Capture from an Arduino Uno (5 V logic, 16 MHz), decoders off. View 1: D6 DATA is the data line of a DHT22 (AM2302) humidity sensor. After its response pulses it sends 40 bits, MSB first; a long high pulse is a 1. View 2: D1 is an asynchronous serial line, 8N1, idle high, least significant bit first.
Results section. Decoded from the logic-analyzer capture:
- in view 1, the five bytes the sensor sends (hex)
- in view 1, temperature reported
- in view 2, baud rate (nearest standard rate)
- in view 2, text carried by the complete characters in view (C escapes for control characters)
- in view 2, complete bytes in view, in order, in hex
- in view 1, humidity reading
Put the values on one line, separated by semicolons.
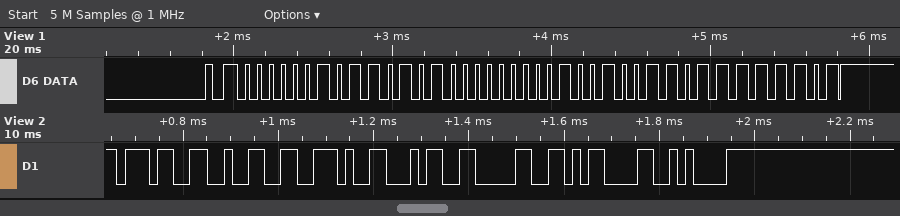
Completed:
02 D4 01 26 FD; 29.4 °C; 57600 baud; "72.40\r\n"; 37 32 2E 34 30 0D 0A; 72.4 %
